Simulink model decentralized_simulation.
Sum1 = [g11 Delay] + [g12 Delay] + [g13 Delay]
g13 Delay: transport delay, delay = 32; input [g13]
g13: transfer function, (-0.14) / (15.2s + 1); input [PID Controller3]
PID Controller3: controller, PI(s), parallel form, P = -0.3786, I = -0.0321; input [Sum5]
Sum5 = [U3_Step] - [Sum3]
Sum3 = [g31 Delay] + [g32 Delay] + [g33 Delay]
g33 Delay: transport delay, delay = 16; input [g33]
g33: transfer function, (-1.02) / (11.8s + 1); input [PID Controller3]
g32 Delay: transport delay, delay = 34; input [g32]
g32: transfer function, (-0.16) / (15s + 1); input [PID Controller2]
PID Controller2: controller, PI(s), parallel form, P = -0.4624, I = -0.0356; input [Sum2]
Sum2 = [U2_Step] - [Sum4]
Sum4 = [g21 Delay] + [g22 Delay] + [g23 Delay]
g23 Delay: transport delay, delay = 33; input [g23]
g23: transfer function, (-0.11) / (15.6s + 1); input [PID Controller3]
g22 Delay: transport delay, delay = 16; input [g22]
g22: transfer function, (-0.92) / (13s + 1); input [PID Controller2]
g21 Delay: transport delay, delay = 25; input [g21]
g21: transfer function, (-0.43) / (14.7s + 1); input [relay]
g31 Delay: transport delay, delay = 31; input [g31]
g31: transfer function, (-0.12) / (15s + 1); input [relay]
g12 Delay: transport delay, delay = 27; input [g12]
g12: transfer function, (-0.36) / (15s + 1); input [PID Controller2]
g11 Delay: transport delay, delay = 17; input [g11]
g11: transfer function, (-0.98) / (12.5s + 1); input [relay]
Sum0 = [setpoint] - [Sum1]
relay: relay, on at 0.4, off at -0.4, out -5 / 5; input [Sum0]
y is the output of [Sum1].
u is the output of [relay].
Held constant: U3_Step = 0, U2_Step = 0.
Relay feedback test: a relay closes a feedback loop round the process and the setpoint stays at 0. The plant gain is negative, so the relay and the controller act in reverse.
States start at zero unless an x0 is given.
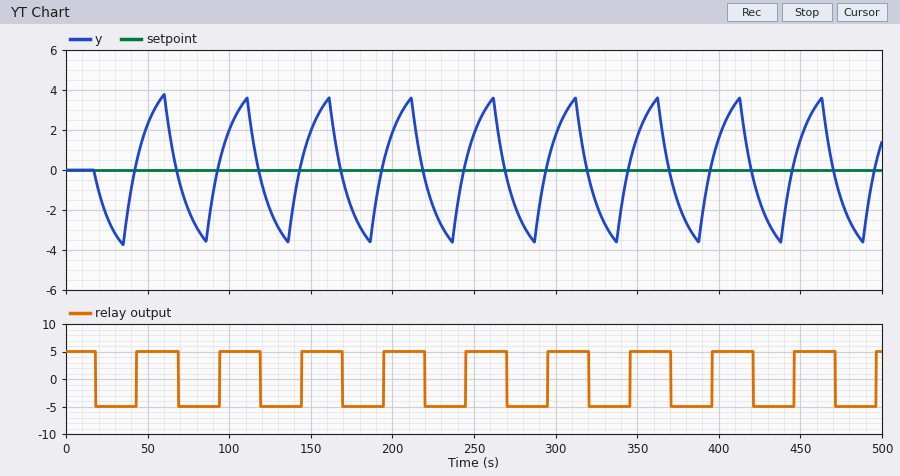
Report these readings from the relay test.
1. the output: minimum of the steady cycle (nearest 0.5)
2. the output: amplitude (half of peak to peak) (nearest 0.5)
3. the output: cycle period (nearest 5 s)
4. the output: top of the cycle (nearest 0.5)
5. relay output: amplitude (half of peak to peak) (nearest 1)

-3.5
3.5
50 s
3.5
5
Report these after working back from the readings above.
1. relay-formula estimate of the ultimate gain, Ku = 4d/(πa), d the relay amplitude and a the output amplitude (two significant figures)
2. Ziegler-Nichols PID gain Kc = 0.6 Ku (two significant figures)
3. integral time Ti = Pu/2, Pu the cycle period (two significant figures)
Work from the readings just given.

1.8
1.1
25 s
